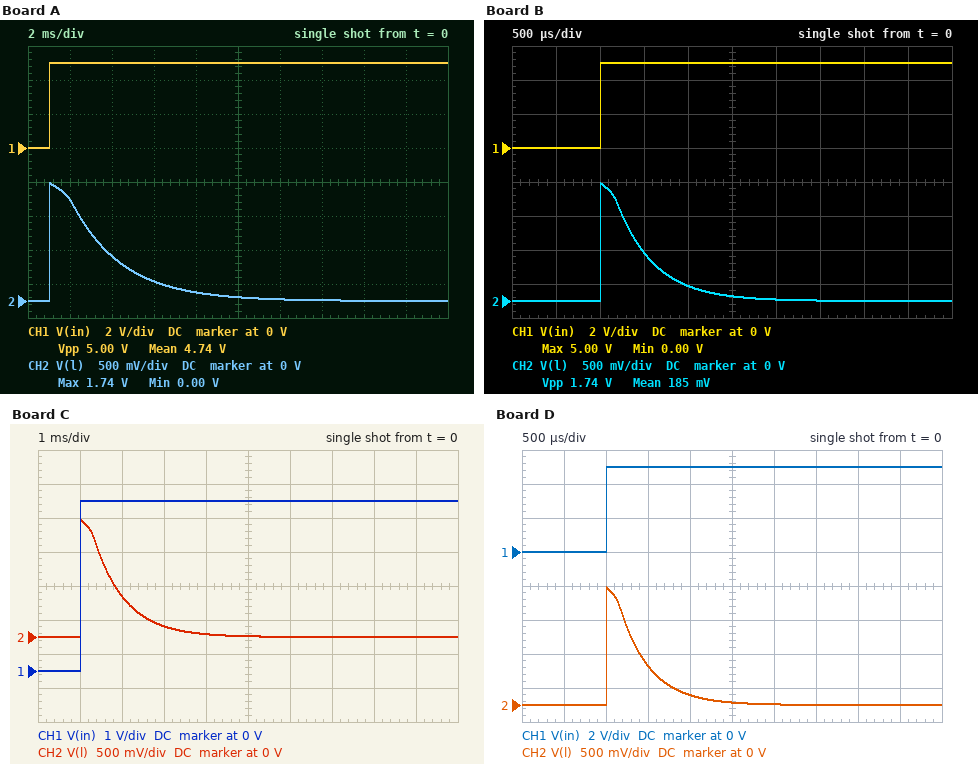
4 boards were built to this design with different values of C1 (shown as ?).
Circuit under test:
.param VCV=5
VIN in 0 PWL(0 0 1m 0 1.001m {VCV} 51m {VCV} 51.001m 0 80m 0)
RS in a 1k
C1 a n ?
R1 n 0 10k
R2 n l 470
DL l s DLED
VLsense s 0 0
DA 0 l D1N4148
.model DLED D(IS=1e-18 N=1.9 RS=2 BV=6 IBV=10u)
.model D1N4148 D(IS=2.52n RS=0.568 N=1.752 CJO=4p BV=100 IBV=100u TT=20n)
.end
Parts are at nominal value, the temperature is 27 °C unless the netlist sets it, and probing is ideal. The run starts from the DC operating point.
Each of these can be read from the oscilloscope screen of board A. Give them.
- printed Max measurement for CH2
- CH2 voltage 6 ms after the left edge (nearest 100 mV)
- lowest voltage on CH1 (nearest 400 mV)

1.74 V
300 mV
0 V
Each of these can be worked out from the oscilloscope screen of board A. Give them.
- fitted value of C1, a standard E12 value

220 nF
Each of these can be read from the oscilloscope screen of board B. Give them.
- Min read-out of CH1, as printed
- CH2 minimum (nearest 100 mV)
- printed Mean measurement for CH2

0.00 V
0 V
185 mV
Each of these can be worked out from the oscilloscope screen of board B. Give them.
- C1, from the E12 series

39 nF
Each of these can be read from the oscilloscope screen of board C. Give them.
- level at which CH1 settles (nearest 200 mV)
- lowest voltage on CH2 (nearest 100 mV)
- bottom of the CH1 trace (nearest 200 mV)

5.0 V
0 V
0 V
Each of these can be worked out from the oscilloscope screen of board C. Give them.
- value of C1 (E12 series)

68 nF
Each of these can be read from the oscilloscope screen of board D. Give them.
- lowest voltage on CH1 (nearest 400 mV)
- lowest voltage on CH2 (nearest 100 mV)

0 V
0 V
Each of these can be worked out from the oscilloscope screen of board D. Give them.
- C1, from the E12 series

33 nF
